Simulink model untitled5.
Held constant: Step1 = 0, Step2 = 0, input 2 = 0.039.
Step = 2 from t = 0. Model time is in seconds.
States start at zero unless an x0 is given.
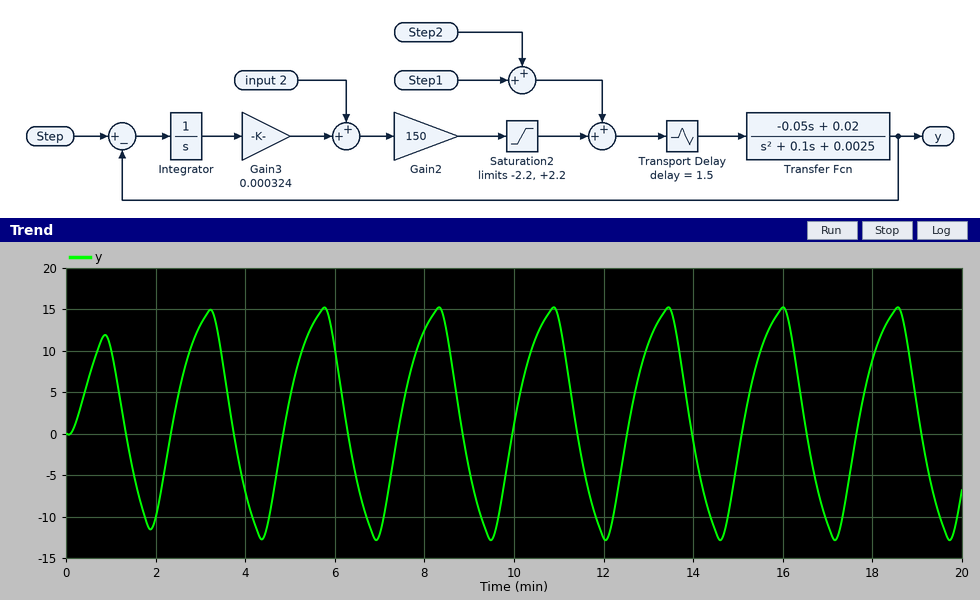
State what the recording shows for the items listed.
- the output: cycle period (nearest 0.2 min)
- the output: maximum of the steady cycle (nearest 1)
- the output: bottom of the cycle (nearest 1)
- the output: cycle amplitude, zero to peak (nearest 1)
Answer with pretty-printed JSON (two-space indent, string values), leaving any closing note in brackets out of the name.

{
  "the output: cycle period": "2.6 min",
  "the output: maximum of the steady cycle": "15",
  "the output: bottom of the cycle": "-13",
  "the output: cycle amplitude, zero to peak": "14"
}
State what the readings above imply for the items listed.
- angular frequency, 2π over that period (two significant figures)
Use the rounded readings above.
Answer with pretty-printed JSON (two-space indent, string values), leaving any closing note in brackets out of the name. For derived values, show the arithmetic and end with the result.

{
  "angular frequency, 2π over that period": "2π / 2.6 = 2.4 rad/min"
}
